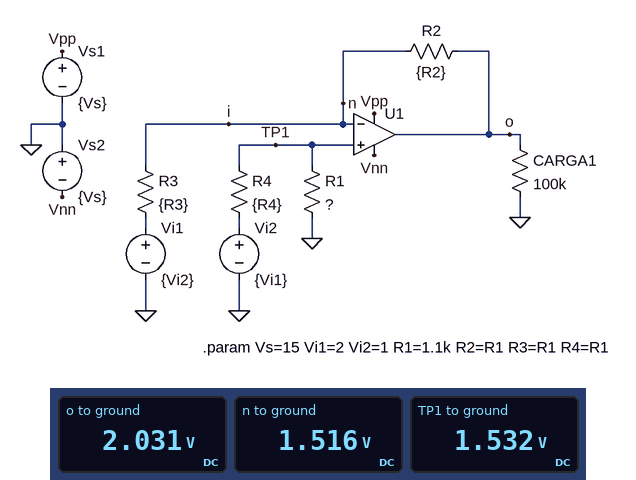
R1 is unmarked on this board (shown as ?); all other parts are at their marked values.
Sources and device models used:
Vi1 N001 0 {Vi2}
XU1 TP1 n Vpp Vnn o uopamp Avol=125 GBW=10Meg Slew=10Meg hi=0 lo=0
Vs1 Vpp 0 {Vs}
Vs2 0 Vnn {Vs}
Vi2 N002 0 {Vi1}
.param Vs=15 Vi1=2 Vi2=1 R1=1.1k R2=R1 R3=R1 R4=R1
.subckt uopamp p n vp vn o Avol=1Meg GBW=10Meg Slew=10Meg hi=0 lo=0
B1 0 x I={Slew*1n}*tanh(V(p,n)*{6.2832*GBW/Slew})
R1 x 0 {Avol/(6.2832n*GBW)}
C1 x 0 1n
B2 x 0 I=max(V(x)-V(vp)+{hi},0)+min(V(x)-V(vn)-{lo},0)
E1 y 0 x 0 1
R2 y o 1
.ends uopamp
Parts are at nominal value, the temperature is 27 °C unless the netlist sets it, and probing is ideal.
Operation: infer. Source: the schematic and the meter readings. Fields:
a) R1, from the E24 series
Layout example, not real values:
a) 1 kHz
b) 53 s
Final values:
a) 3.6 kΩ
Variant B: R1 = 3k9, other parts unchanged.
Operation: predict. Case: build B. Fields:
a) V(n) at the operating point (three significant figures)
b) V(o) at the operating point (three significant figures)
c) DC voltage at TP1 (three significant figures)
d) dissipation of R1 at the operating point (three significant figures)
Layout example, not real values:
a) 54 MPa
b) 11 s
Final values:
a) 1.54 V
b) 2.09 V
c) 1.56 V
d) 624 µW
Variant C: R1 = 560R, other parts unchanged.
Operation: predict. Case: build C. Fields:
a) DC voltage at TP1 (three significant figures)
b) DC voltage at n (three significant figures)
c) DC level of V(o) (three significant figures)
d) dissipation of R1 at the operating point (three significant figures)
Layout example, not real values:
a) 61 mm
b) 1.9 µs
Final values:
a) 675 mV
b) 672 mV
c) 344 mV
d) 813 µW
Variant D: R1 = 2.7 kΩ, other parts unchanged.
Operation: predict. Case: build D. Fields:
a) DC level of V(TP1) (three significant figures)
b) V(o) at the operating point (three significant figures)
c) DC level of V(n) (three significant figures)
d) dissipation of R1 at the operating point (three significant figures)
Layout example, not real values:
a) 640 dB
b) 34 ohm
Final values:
a) 1.42 V
b) 1.81 V
c) 1.41 V
d) 748 µW
